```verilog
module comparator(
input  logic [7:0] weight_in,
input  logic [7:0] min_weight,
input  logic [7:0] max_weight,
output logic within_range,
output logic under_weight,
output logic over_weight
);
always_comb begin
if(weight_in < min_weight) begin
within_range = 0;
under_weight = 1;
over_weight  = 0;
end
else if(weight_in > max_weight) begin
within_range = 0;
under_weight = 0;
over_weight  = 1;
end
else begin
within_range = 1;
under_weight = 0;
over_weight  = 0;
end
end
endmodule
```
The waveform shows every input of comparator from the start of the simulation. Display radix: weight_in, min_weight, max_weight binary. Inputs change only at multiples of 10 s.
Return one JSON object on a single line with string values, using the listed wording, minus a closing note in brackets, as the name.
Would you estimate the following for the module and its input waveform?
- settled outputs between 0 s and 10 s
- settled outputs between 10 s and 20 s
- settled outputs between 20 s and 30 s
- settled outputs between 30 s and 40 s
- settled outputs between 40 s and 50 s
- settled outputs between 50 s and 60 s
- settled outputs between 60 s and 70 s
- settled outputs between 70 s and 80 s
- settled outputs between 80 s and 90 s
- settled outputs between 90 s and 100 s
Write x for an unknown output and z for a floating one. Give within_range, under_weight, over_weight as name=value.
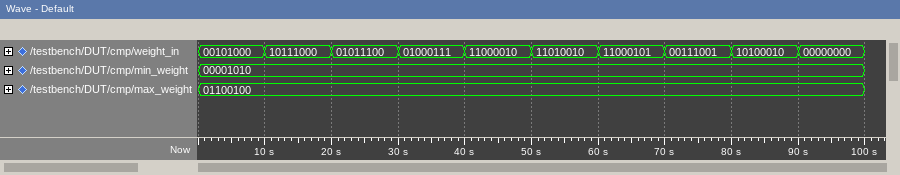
{"settled outputs between 0 s and 10 s": "within_range=1, under_weight=0, over_weight=0", "settled outputs between 10 s and 20 s": "within_range=0, under_weight=0, over_weight=1", "settled outputs between 20 s and 30 s": "within_range=1, under_weight=0, over_weight=0", "settled outputs between 30 s and 40 s": "within_range=1, under_weight=0, over_weight=0", "settled outputs between 40 s and 50 s": "within_range=0, under_weight=0, over_weight=1", "settled outputs between 50 s and 60 s": "within_range=0, under_weight=0, over_weight=1", "settled outputs between 60 s and 70 s": "within_range=0, under_weight=0, over_weight=1", "settled outputs between 70 s and 80 s": "within_range=1, under_weight=0, over_weight=0", "settled outputs between 80 s and 90 s": "within_range=0, under_weight=0, over_weight=1", "settled outputs between 90 s and 100 s": "within_range=0, under_weight=1, over_weight=0"}
